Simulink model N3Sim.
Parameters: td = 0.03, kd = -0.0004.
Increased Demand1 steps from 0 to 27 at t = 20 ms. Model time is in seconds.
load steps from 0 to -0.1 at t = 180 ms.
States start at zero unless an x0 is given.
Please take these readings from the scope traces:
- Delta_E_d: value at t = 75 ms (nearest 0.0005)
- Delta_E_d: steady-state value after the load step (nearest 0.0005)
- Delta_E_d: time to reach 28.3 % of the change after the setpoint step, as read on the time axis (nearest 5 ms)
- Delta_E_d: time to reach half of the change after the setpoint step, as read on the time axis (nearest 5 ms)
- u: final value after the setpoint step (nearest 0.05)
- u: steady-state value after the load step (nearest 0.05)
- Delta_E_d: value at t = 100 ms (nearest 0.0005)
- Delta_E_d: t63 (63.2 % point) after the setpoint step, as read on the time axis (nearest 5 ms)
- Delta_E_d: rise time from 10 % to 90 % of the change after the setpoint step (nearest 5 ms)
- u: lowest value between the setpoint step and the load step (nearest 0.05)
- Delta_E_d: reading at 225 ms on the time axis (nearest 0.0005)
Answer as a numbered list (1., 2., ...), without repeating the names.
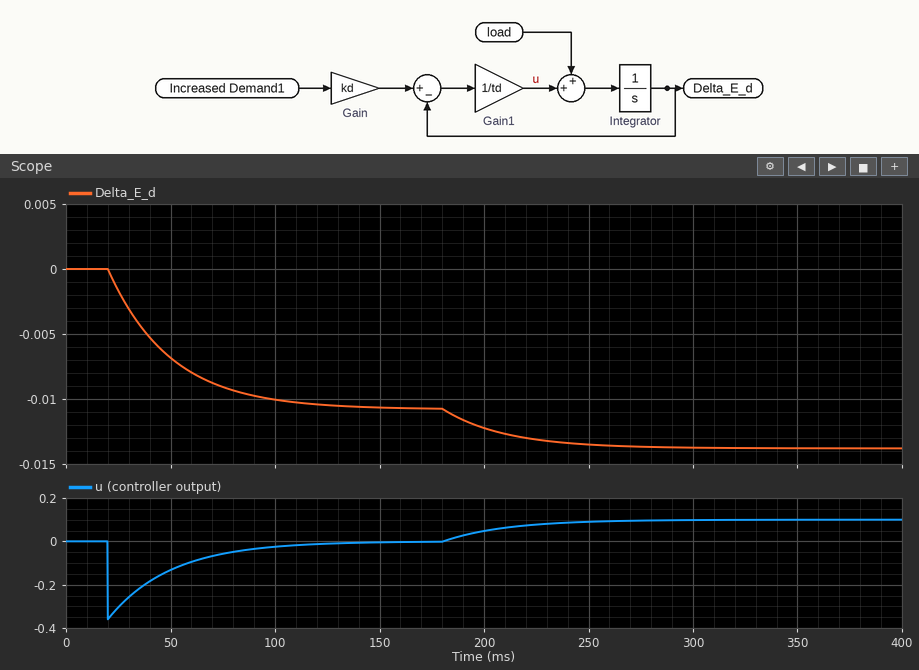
1. -0.0090
2. -0.0140
3. 30 ms
4. 40 ms
5. 0.00
6. 0.10
7. -0.0100
8. 50 ms
9. 65 ms
10. -0.35
11. -0.0130
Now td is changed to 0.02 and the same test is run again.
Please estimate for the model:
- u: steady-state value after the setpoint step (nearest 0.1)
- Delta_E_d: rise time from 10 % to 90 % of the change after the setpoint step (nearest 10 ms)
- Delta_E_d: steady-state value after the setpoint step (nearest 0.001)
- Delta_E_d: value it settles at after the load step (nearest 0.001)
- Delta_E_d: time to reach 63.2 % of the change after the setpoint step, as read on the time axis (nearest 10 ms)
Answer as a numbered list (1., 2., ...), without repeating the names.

1. 0.0
2. 40 ms
3. -0.011
4. -0.013
5. 40 ms
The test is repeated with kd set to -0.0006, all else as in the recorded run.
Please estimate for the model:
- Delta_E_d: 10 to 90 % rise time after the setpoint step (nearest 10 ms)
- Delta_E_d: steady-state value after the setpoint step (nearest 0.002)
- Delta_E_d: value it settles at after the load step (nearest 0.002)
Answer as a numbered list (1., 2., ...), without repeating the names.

1. 70 ms
2. -0.016
3. -0.020
